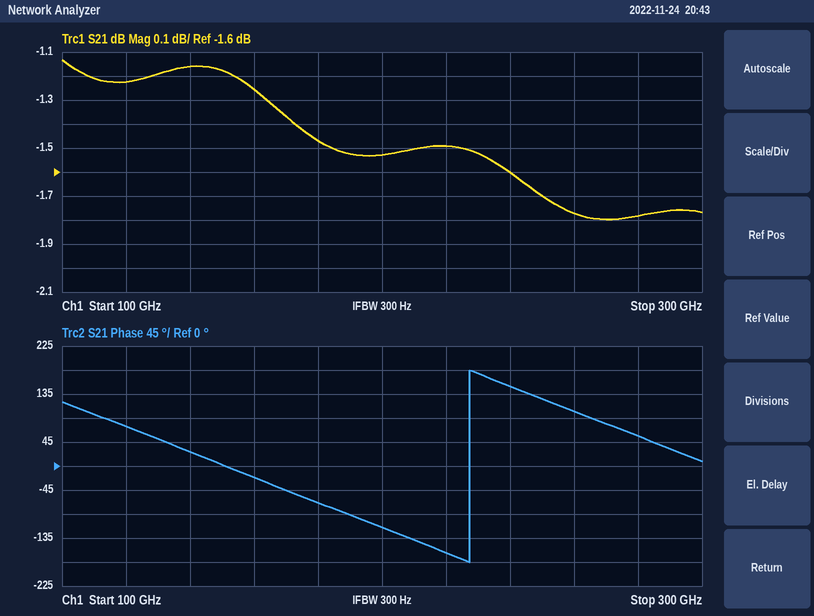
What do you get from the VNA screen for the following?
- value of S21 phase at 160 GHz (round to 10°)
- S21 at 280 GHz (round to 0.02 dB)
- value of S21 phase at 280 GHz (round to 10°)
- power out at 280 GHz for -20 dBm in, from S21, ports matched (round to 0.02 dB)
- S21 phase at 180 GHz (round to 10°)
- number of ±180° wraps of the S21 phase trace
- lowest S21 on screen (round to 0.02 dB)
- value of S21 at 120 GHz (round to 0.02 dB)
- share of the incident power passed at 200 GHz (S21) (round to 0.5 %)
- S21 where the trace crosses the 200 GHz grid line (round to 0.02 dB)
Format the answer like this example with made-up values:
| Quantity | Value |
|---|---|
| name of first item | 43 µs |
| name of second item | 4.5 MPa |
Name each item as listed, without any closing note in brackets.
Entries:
| Quantity | Value |
|---|---|
| value of S21 phase at 160 GHz | -20° |
| S21 at 280 GHz | -1.78 dB |
| value of S21 phase at 280 GHz | 60° |
| power out at 280 GHz for -20 dBm in, from S21, ports matched | -21.78 dBm |
| S21 phase at 180 GHz | -70° |
| number of ±180° wraps of the S21 phase trace | 1 |
| lowest S21 on screen | -1.80 dB |
| value of S21 at 120 GHz | -1.22 dB |
| share of the incident power passed at 200 GHz (S21) | 70.5 % |
| S21 where the trace crosses the 200 GHz grid line | -1.52 dB |
